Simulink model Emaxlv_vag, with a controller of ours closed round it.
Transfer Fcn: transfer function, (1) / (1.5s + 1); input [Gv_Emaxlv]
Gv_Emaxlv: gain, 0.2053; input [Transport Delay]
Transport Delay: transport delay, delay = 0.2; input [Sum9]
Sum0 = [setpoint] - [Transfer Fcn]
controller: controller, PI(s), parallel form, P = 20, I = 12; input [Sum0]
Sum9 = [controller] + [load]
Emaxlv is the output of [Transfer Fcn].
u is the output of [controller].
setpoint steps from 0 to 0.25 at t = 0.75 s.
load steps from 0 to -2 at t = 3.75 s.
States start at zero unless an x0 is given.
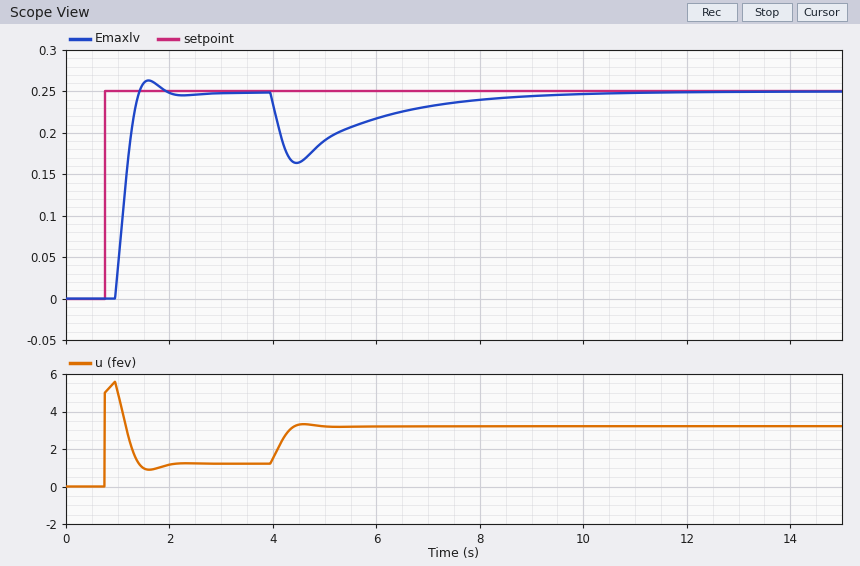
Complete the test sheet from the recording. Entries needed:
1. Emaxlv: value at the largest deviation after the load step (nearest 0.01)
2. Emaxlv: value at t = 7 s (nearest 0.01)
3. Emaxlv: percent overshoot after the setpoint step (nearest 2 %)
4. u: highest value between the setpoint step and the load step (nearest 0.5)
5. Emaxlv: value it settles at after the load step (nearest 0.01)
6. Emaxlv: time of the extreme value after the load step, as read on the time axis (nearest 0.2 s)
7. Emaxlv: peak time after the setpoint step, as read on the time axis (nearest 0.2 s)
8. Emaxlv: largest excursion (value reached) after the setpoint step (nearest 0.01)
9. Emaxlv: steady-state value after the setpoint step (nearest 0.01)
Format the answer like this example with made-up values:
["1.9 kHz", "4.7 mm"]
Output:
["0.16", "0.23", "6 %", "5.5", "0.25", "4.4 s", "1.6 s", "0.26", "0.25"]
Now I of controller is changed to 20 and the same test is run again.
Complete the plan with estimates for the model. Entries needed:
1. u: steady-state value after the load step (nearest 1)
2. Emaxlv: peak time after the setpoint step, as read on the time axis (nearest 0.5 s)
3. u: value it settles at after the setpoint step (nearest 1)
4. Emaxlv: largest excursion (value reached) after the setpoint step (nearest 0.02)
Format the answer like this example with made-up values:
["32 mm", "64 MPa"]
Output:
["3", "1.5 s", "1", "0.30"]
